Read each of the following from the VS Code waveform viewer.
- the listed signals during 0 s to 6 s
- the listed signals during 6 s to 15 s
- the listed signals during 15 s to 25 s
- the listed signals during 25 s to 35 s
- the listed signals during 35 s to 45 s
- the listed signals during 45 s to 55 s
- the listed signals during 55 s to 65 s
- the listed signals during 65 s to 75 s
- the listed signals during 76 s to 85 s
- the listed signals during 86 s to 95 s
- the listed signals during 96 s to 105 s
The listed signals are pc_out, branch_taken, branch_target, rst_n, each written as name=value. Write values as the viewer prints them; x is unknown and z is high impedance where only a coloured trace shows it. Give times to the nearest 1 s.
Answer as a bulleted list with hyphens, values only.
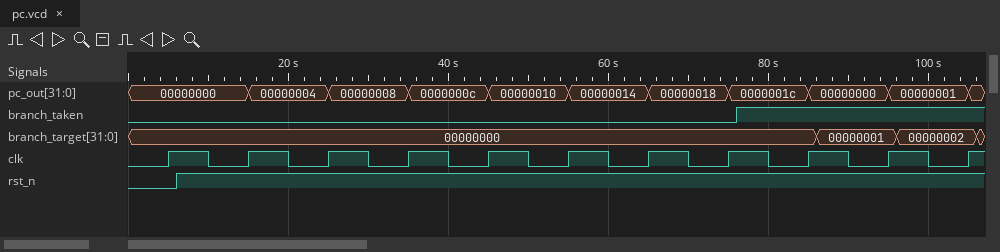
- pc_out=00000000, branch_taken=0, branch_target=00000000, rst_n=0
- pc_out=00000000, branch_taken=0, branch_target=00000000, rst_n=1
- pc_out=00000004, branch_taken=0, branch_target=00000000, rst_n=1
- pc_out=00000008, branch_taken=0, branch_target=00000000, rst_n=1
- pc_out=0000000c, branch_taken=0, branch_target=00000000, rst_n=1
- pc_out=00000010, branch_taken=0, branch_target=00000000, rst_n=1
- pc_out=00000014, branch_taken=0, branch_target=00000000, rst_n=1
- pc_out=00000018, branch_taken=0, branch_target=00000000, rst_n=1
- pc_out=0000001c, branch_taken=1, branch_target=00000000, rst_n=1
- pc_out=00000000, branch_taken=1, branch_target=00000001, rst_n=1
- pc_out=00000001, branch_taken=1, branch_target=00000002, rst_n=1
